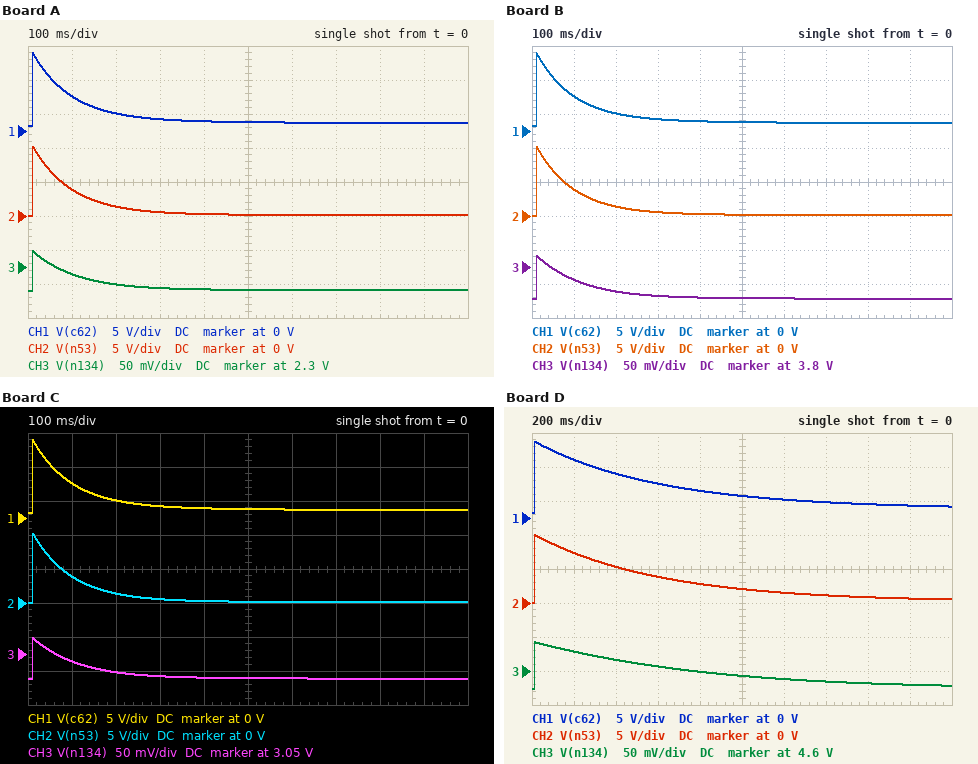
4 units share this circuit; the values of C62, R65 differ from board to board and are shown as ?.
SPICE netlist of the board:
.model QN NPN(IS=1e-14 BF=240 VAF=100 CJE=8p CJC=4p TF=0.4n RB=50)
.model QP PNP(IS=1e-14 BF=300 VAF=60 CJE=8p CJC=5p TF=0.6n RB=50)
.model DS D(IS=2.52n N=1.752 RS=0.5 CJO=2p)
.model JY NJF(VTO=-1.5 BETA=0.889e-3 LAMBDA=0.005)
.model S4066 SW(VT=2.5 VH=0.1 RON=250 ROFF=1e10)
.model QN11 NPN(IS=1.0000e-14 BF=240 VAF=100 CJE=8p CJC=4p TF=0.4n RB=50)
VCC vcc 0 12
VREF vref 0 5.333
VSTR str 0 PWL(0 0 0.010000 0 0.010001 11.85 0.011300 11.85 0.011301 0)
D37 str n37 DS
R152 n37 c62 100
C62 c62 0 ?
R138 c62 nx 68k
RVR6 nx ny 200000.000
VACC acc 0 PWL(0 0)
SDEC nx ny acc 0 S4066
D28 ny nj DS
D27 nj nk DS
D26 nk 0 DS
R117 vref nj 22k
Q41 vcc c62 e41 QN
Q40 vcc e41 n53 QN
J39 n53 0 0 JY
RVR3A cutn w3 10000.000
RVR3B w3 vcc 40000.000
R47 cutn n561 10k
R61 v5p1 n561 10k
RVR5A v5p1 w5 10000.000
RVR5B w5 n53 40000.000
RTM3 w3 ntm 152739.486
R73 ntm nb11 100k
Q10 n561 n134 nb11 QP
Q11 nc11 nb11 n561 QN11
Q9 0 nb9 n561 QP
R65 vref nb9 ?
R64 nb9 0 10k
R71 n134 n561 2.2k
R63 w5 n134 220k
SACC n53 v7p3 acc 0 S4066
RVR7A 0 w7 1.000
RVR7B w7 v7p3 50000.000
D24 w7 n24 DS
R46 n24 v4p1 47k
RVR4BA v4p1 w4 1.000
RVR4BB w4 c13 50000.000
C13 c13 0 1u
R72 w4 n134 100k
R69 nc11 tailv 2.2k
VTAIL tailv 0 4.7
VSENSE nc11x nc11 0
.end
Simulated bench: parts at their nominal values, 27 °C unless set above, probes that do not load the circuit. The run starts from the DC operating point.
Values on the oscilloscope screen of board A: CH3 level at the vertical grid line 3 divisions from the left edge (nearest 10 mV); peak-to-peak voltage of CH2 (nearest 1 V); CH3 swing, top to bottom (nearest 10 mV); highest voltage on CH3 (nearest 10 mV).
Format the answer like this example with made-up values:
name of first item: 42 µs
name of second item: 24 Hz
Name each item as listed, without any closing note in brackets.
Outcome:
CH3 level at the vertical grid line 3 divisions from the left edge: 2.27 V
peak-to-peak voltage of CH2: 10 V
CH3 swing, top to bottom: 60 mV
highest voltage on CH3: 2.32 V
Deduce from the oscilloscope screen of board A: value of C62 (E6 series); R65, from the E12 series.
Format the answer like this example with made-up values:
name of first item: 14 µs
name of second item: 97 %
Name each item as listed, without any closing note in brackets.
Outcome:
value of C62: 330 nF
R65, from the E12 series: 22 kΩ
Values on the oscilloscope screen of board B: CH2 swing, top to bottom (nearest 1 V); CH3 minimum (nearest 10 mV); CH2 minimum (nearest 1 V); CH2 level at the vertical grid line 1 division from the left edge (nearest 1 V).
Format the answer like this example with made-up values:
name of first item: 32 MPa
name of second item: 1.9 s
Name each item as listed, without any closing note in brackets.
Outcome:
CH2 swing, top to bottom: 10 V
CH3 minimum: 3.75 V
CH2 minimum: 0 V
CH2 level at the vertical grid line 1 division from the left edge: 4 V
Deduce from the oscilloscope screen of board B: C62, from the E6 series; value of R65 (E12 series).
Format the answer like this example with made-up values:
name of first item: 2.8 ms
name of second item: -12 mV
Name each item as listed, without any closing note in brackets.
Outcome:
C62, from the E6 series: 330 nF
value of R65: 6.8 kΩ
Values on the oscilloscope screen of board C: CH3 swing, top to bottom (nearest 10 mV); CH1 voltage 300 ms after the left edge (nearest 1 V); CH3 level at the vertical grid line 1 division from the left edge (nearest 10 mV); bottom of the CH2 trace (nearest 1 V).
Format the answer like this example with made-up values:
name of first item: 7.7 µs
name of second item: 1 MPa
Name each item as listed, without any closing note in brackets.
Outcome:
CH3 swing, top to bottom: 60 mV
CH1 voltage 300 ms after the left edge: 2 V
CH3 level at the vertical grid line 1 division from the left edge: 3.04 V
bottom of the CH2 trace: 0 V
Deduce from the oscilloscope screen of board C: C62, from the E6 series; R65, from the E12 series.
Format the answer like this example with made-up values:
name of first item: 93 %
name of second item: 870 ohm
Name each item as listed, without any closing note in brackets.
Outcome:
C62, from the E6 series: 330 nF
R65, from the E12 series: 12 kΩ
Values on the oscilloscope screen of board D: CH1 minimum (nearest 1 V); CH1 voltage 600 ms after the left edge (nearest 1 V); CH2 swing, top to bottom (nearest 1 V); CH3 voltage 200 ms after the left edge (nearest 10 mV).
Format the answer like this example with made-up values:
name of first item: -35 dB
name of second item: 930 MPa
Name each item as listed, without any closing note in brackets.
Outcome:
CH1 minimum: 1 V
CH1 voltage 600 ms after the left edge: 5 V
CH2 swing, top to bottom: 10 V
CH3 voltage 200 ms after the left edge: 4.63 V
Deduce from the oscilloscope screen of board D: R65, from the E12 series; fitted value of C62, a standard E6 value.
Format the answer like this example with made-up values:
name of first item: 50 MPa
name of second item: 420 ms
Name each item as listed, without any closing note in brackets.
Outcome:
R65, from the E12 series: 3.3 kΩ
fitted value of C62, a standard E6 value: 2.2 µF
